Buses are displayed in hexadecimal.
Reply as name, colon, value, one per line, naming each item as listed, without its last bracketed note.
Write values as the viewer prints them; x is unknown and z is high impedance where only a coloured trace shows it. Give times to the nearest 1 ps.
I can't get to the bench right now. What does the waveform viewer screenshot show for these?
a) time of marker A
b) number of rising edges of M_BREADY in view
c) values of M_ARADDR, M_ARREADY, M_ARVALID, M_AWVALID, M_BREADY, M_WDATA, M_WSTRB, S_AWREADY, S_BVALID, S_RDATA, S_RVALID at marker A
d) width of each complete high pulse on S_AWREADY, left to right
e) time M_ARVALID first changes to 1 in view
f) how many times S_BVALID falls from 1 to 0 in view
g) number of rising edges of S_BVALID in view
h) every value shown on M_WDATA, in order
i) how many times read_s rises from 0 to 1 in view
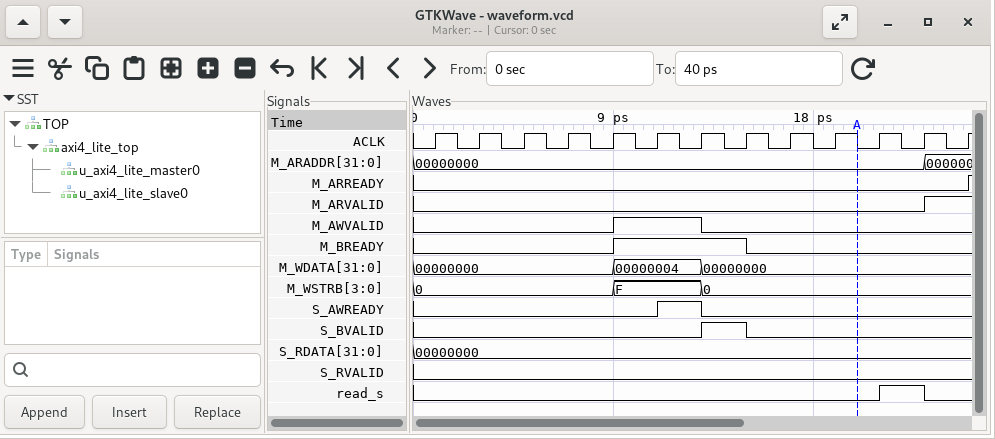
time of marker A: 20 ps
number of rising edges of M_BREADY in view: 1
values of M_ARADDR, M_ARREADY, M_ARVALID, M_AWVALID, M_BREADY, M_WDATA, M_WSTRB, S_AWREADY, S_BVALID, S_RDATA, S_RVALID at marker A: M_ARADDR=00000000, M_ARREADY=0, M_ARVALID=0, M_AWVALID=0, M_BREADY=0, M_WDATA=00000000, M_WSTRB=0, S_AWREADY=0, S_BVALID=0, S_RDATA=00000000, S_RVALID=0
width of each complete high pulse on S_AWREADY, left to right: 2 ps
time M_ARVALID first changes to 1 in view: 23 ps
how many times S_BVALID falls from 1 to 0 in view: 1
number of rising edges of S_BVALID in view: 1
every value shown on M_WDATA, in order: 00000000, 00000004, 00000000
how many times read_s rises from 0 to 1 in view: 1
